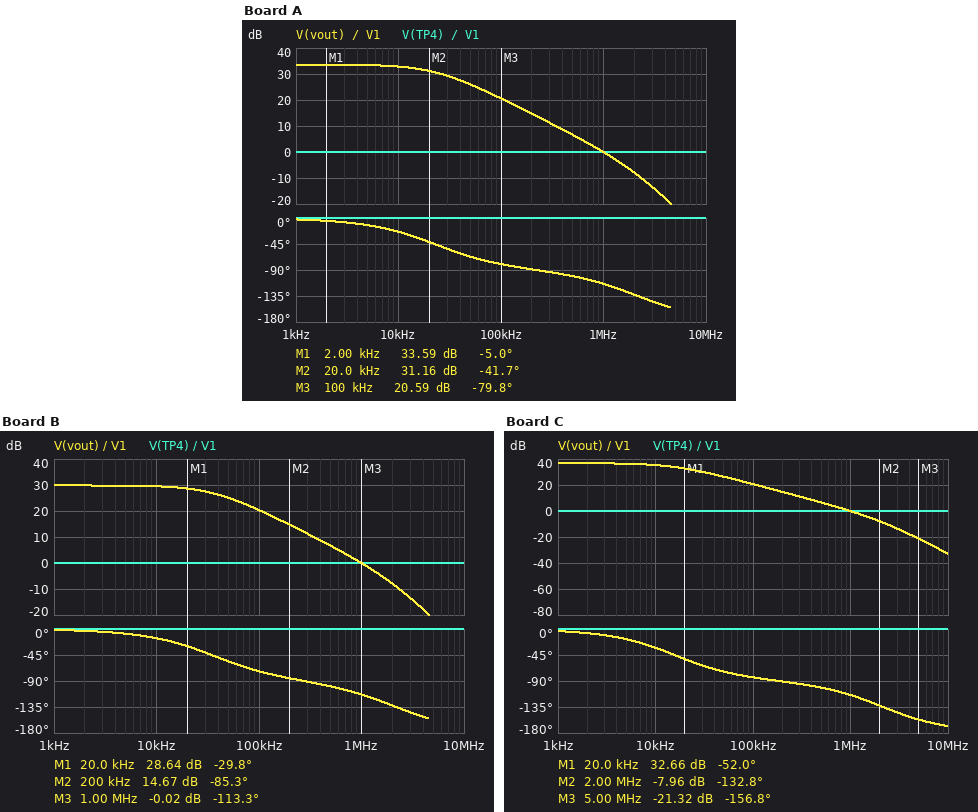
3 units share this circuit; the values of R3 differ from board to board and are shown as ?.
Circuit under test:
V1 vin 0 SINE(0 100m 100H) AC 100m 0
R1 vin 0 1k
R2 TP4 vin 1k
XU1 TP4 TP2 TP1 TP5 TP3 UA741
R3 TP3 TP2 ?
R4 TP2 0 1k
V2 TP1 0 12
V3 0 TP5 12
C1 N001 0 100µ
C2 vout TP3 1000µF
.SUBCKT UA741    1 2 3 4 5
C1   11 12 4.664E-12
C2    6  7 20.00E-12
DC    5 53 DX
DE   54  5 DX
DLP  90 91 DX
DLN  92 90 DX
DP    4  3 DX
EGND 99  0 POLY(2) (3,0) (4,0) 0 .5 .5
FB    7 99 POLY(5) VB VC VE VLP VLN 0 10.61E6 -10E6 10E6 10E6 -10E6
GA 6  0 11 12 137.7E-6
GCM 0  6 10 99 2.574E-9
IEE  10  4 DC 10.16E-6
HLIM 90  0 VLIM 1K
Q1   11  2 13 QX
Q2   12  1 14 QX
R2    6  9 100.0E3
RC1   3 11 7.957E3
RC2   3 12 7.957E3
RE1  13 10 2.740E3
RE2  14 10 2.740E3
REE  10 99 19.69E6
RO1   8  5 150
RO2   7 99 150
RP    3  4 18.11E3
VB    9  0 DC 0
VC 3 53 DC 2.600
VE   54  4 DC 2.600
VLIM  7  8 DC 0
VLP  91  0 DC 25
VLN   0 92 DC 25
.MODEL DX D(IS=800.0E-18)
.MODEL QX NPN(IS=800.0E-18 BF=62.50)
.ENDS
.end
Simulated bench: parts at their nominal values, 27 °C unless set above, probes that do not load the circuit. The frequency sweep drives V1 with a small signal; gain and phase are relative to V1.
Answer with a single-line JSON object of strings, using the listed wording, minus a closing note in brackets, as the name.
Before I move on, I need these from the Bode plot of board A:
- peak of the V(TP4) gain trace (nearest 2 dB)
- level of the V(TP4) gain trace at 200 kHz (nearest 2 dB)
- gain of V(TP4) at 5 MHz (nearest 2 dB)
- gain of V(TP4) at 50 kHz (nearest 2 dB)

{"peak of the V(TP4) gain trace": "0 dB", "level of the V(TP4) gain trace at 200 kHz": "0 dB", "gain of V(TP4) at 5 MHz": "0 dB", "gain of V(TP4) at 50 kHz": "0 dB"}
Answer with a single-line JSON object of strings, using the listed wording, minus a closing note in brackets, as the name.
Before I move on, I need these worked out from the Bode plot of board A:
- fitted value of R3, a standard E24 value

{"fitted value of R3, a standard E24 value": "47 kΩ"}
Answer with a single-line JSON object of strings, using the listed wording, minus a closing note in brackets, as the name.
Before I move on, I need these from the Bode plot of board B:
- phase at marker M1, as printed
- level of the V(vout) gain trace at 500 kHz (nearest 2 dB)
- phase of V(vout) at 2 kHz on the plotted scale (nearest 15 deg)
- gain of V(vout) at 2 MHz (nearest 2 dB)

{"phase at marker M1, as printed": "-29.8 deg", "level of the V(vout) gain trace at 500 kHz": "6 dB", "phase of V(vout) at 2 kHz on the plotted scale": "0 deg", "gain of V(vout) at 2 MHz": "-8 dB"}
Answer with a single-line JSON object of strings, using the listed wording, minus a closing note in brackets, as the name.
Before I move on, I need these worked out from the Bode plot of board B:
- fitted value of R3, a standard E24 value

{"fitted value of R3, a standard E24 value": "30 kΩ"}
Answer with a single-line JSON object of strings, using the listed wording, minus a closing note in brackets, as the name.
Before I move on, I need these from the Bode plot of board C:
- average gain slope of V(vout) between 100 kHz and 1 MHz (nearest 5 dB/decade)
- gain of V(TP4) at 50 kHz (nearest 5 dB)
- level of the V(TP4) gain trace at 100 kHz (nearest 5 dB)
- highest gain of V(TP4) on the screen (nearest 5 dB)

{"average gain slope of V(vout) between 100 kHz and 1 MHz": "-20 dB/decade", "gain of V(TP4) at 50 kHz": "0 dB", "level of the V(TP4) gain trace at 100 kHz": "0 dB", "highest gain of V(TP4) on the screen": "0 dB"}
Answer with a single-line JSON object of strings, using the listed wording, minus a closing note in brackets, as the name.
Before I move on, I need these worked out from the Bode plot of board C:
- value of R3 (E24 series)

{"value of R3": "68 kΩ"}
